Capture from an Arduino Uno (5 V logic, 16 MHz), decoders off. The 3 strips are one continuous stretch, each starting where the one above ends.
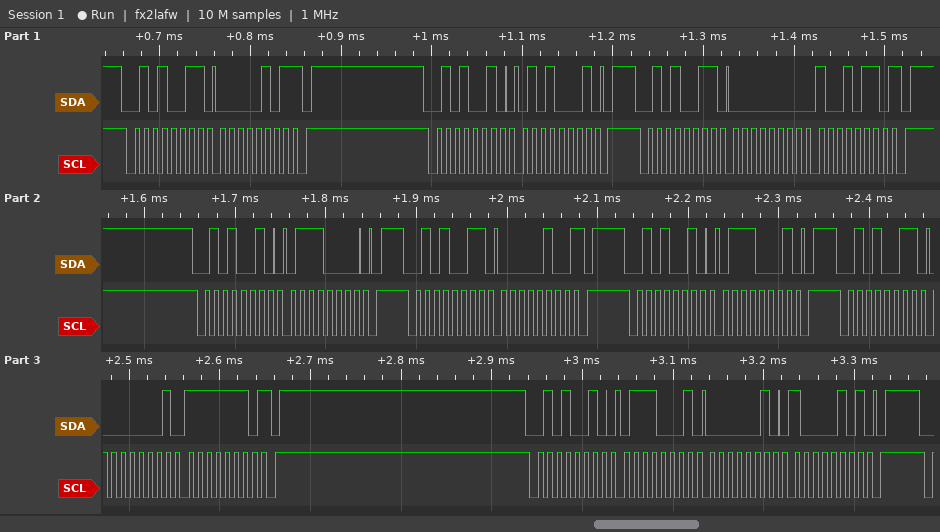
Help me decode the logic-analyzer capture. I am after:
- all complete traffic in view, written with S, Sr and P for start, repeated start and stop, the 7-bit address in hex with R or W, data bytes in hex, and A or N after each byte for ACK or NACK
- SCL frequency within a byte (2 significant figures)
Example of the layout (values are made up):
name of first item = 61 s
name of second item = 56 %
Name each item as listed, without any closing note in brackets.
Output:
all complete traffic in view, written with S, Sr and P for start, repeated start and stop, the 7-bit address in hex with R or W, data bytes in hex, and A or N after each byte for ACK or NACK = S 29R A 05 N P S 29W A 51 A P S 29R A 00 A 96 N P S 29W A 70 A P S 29R A 04 N P S 29W A 71 A P S 29R A 01 A FE N P S 29W A 71 A 02 A 85 A P
SCL frequency within a byte = 100 kHz
